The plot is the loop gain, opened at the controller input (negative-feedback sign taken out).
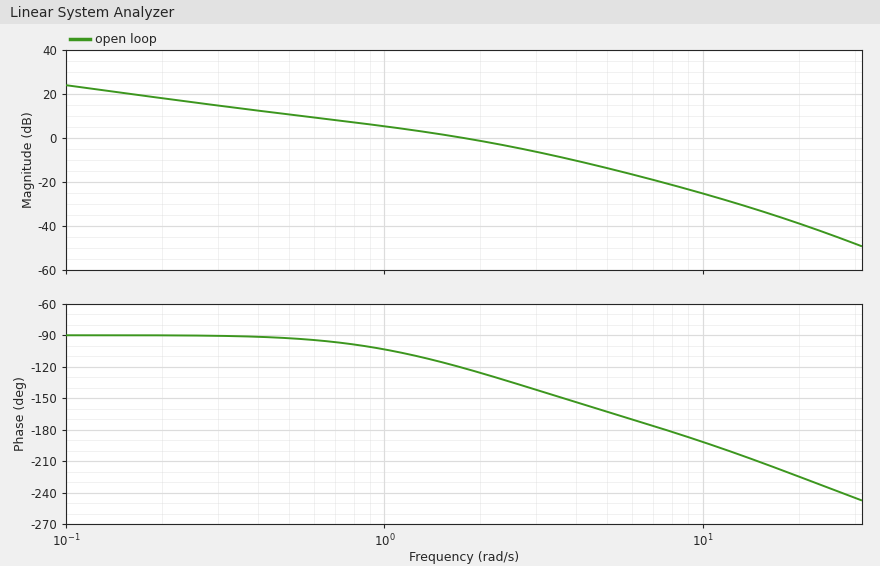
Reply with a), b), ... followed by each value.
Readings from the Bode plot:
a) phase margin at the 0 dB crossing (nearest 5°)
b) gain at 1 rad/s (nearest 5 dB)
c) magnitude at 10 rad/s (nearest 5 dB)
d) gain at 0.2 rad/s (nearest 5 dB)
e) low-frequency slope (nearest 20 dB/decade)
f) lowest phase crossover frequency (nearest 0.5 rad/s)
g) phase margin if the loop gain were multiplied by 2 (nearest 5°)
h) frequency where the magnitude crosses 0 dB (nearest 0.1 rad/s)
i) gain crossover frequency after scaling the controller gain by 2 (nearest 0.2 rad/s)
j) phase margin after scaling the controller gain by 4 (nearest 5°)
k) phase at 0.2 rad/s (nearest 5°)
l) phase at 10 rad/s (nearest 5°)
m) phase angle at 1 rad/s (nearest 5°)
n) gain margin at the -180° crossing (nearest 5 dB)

a) 60°
b) 5 dB
c) -25 dB
d) 20 dB
e) -20 dB/decade
f) 7.5 rad/s
g) 40°
h) 1.8 rad/s
i) 3.0 rad/s
j) 20°
k) -90°
l) -190°
m) -105°
n) 20 dB
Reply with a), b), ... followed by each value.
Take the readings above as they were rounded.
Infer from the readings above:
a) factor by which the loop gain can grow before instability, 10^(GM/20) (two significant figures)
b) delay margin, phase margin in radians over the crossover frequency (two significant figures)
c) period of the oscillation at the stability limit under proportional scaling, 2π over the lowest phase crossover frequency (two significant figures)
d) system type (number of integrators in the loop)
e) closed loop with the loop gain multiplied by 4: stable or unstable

a) 10
b) 0.58 s
c) 0.84 s
d) 1
e) stable
